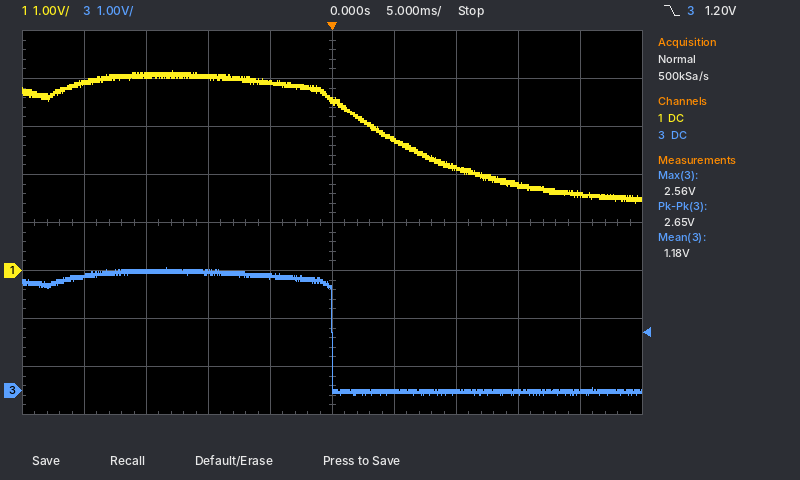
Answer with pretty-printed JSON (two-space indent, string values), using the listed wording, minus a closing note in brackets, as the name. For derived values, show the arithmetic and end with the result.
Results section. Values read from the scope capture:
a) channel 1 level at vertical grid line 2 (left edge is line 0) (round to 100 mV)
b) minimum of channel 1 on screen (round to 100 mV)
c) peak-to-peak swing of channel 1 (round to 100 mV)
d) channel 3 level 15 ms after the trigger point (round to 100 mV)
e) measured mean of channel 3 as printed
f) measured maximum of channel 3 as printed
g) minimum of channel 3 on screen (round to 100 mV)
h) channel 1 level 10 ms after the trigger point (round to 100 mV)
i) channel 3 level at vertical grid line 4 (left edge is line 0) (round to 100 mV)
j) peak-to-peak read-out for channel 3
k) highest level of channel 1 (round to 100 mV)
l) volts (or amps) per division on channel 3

{
  "channel 1 level at vertical grid line 2 (left edge is line 0)": "4.1 V",
  "minimum of channel 1 on screen": "1.4 V",
  "peak-to-peak swing of channel 1": "4.2 V − (1.4 V) = 2.8 V",
  "channel 3 level 15 ms after the trigger point": "0.0 V",
  "measured mean of channel 3 as printed": "1.18 V",
  "measured maximum of channel 3 as printed": "2.56 V",
  "minimum of channel 3 on screen": "-100 mV",
  "channel 1 level 10 ms after the trigger point": "2.1 V",
  "channel 3 level at vertical grid line 4 (left edge is line 0)": "2.4 V",
  "peak-to-peak read-out for channel 3": "2.65 V",
  "highest level of channel 1": "4.2 V",
  "volts (or amps) per division on channel 3": "1 V"
}
